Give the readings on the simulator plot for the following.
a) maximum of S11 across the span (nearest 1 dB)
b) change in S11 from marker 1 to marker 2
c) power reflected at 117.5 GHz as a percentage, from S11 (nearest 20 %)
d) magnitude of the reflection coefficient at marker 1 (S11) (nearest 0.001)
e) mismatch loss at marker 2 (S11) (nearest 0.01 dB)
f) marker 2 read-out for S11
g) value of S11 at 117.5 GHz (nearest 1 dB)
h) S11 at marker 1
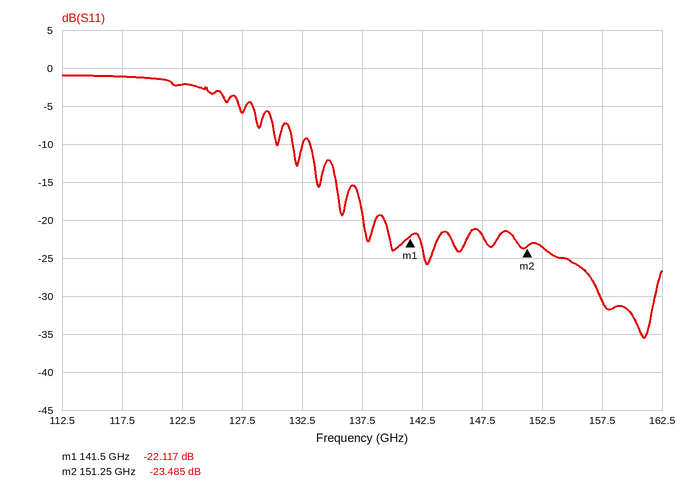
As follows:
-1 dB
-1.368 dB
80 %
0.078
0.02 dB
-23.485 dB
-1 dB
-22.117 dB
